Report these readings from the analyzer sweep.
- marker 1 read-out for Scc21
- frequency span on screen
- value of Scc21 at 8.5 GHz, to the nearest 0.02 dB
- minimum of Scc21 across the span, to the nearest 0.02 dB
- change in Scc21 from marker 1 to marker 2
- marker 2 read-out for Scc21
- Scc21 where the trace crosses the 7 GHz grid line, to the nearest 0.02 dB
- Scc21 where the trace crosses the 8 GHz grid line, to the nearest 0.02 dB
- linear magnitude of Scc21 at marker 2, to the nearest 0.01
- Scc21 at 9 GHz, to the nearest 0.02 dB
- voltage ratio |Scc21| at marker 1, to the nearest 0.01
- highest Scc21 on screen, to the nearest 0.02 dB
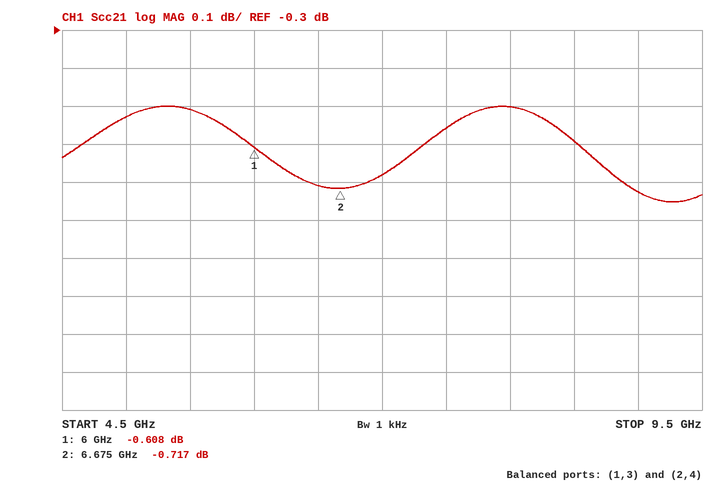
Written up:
-0.608 dB
5 GHz
-0.60 dB
-0.76 dB
-0.109 dB
-0.717 dB
-0.68 dB
-0.50 dB
0.92
-0.72 dB
0.93
-0.50 dB
